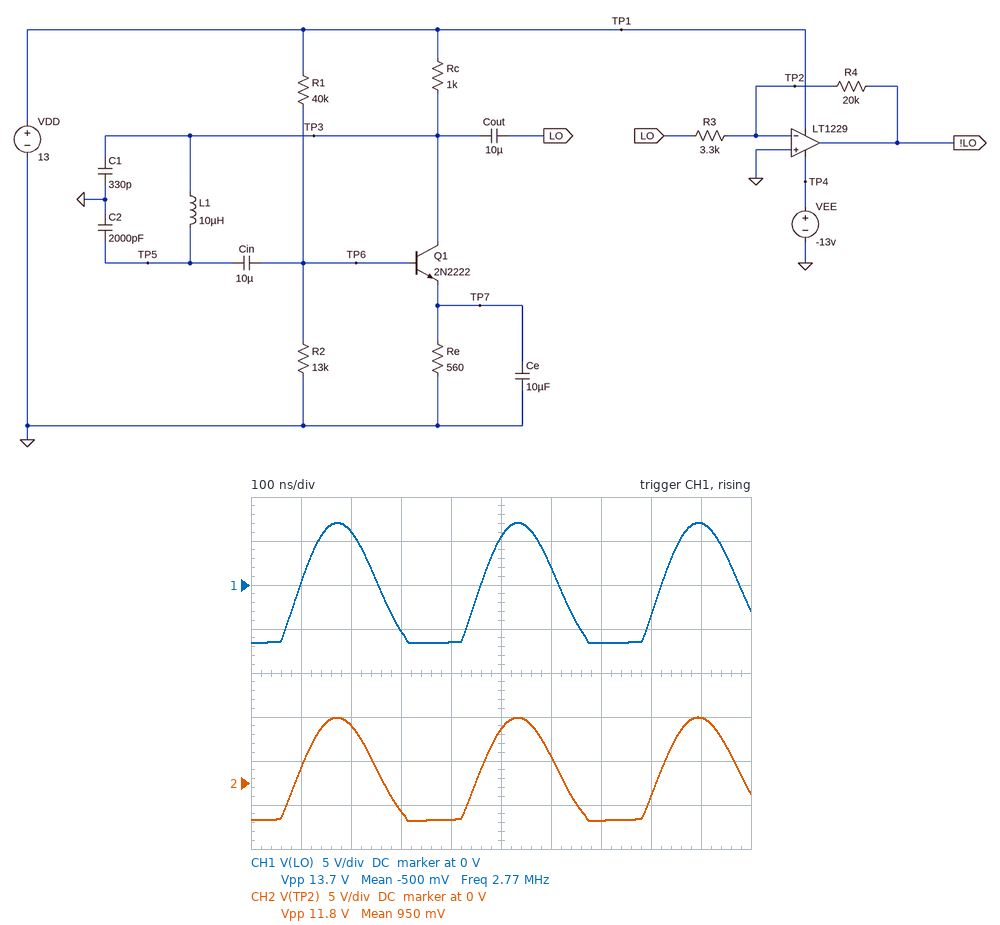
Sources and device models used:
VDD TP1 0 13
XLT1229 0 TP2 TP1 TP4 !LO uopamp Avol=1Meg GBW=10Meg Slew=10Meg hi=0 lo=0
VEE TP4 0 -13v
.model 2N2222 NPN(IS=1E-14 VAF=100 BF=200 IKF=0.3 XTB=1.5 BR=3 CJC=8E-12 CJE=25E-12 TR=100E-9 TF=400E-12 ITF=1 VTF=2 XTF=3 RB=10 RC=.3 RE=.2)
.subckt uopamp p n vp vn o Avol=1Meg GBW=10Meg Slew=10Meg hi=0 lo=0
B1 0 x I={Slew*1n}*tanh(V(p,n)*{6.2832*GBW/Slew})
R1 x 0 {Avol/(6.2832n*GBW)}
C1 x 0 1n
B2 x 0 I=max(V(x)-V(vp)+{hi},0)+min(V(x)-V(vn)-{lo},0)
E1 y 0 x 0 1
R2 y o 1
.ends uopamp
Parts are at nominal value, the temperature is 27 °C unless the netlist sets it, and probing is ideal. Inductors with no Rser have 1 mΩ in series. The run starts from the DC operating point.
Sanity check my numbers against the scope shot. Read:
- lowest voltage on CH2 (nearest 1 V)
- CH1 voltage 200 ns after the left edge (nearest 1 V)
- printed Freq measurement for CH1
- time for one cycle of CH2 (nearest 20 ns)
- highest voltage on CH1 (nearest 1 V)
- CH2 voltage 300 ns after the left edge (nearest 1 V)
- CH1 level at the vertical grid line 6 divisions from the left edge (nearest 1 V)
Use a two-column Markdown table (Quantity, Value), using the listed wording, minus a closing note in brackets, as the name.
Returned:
| Quantity | Value |
|---|---|
| lowest voltage on CH2 | -4 V |
| CH1 voltage 200 ns after the left edge | 6 V |
| printed Freq measurement for CH1 | 2.77 MHz |
| time for one cycle of CH2 | 360 ns |
| highest voltage on CH1 | 7 V |
| CH2 voltage 300 ns after the left edge | -3 V |
| CH1 level at the vertical grid line 6 divisions from the left edge | 2 V |
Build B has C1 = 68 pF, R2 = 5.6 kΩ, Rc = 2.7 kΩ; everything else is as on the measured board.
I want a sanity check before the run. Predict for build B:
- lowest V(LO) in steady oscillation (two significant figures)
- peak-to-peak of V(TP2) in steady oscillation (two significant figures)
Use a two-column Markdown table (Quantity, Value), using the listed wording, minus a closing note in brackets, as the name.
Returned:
| Quantity | Value |
|---|---|
| lowest V(LO) in steady oscillation | -7.7 V |
| peak-to-peak of V(TP2) in steady oscillation | 13 V |
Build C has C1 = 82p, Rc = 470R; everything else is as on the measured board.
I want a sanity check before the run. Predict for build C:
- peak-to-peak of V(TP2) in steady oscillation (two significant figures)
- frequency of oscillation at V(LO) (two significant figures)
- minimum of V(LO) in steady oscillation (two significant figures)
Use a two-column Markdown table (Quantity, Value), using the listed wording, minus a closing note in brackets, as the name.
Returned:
| Quantity | Value |
|---|---|
| peak-to-peak of V(TP2) in steady oscillation | 7.3 V |
| frequency of oscillation at V(LO) | 5.2 MHz |
| minimum of V(LO) in steady oscillation | -4.9 V |
